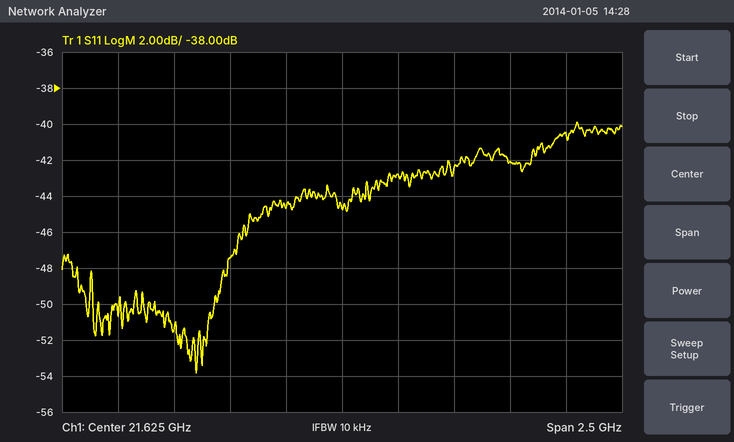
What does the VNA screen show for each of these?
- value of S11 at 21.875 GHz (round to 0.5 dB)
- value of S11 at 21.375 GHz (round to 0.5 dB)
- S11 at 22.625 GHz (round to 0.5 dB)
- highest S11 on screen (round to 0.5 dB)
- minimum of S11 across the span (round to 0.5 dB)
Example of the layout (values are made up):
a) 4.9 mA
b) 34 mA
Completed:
a) -43.0 dB
b) -44.5 dB
c) -40.5 dB
d) -40.0 dB
e) -54.0 dB
